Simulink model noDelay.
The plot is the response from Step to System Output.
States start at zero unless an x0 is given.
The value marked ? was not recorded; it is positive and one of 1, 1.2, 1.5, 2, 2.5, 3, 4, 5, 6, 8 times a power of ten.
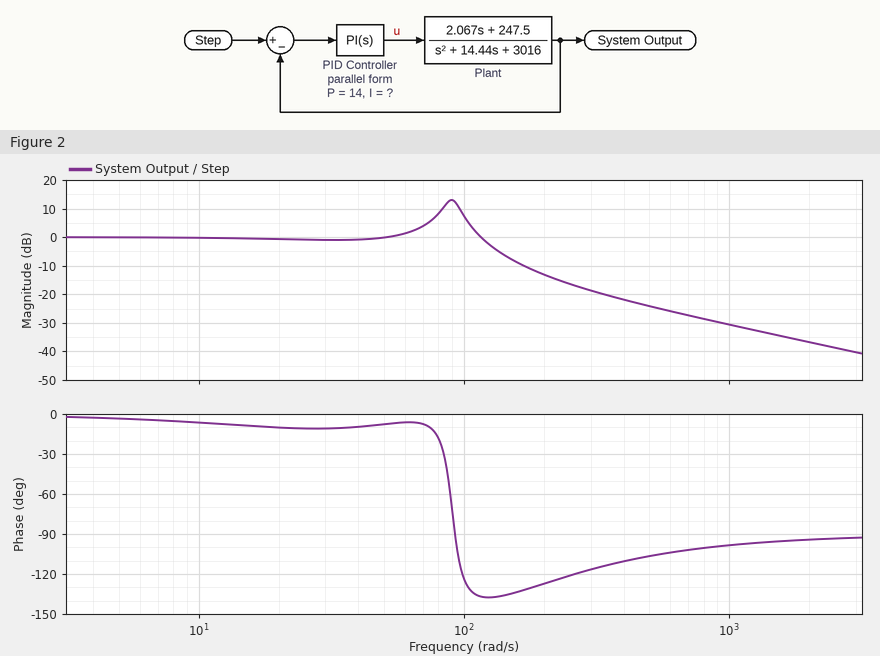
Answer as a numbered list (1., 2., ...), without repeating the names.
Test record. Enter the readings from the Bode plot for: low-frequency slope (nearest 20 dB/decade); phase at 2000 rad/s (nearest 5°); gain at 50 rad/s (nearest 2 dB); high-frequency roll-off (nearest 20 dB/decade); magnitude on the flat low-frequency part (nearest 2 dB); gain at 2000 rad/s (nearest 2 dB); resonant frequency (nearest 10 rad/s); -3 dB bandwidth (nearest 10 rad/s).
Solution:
1. 0 dB/decade
2. -95°
3. 0 dB
4. -20 dB/decade
5. 0 dB
6. -36 dB
7. 90 rad/s
8. 130 rad/s
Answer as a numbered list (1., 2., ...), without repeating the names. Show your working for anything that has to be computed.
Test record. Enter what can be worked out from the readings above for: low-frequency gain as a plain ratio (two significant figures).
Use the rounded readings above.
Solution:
1. 10^(0 / 20) = 1.0
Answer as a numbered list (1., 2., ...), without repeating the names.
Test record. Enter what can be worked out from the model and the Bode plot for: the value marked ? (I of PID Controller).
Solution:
1. 1000
